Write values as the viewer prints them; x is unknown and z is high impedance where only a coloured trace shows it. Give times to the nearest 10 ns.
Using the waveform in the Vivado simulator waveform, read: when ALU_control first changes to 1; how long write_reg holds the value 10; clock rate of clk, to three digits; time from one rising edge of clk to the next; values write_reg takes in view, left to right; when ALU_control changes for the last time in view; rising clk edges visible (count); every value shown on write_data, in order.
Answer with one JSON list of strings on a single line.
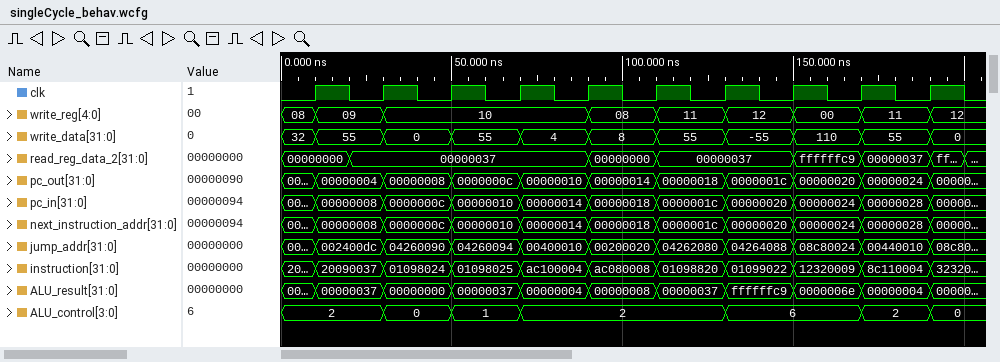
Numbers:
["50 ns", "60 ns", "50.0 MHz", "20 ns", "08, 09, 10, 08, 11, 12, 00, 11, 12", "190 ns", "10", "32, 55, 0, 55, 4, 8, 55, -55, 110, 55, 0"]
